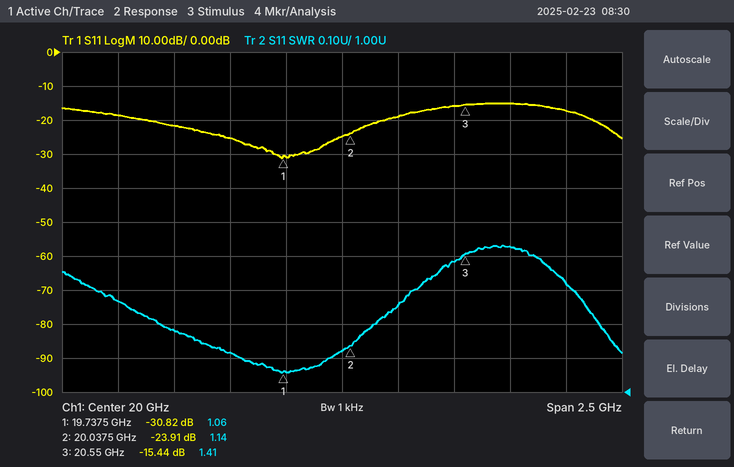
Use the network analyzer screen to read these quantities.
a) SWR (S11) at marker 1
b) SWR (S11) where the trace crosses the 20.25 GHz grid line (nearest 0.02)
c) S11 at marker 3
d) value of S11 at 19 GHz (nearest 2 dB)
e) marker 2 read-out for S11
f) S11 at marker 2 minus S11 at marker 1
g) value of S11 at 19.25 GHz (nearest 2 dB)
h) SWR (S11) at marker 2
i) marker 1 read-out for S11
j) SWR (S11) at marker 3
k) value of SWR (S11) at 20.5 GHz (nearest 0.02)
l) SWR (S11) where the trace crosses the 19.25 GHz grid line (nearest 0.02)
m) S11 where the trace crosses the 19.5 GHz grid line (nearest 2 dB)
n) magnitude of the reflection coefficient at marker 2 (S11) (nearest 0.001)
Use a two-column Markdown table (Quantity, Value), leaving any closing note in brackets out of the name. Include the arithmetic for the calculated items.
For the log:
| Quantity | Value |
|---|---|
| SWR (S11) at marker 1 | 1.06 |
| SWR (S11) where the trace crosses the 20.25 GHz grid line | 1.26 |
| S11 at marker 3 | -15.44 dB |
| value of S11 at 19 GHz | -18 dB |
| marker 2 read-out for S11 | -23.91 dB |
| S11 at marker 2 minus S11 at marker 1 | -23.91 − (-30.82) = 6.91 dB |
| value of S11 at 19.25 GHz | -22 dB |
| SWR (S11) at marker 2 | 1.14 |
| marker 1 read-out for S11 | -30.82 dB |
| SWR (S11) at marker 3 | 1.41 |
| value of SWR (S11) at 20.5 GHz | 1.38 |
| SWR (S11) where the trace crosses the 19.25 GHz grid line | 1.18 |
| S11 where the trace crosses the 19.5 GHz grid line | -26 dB |
| magnitude of the reflection coefficient at marker 2 (S11) | 10^(-23.91/20) ≈ 0.064 |
